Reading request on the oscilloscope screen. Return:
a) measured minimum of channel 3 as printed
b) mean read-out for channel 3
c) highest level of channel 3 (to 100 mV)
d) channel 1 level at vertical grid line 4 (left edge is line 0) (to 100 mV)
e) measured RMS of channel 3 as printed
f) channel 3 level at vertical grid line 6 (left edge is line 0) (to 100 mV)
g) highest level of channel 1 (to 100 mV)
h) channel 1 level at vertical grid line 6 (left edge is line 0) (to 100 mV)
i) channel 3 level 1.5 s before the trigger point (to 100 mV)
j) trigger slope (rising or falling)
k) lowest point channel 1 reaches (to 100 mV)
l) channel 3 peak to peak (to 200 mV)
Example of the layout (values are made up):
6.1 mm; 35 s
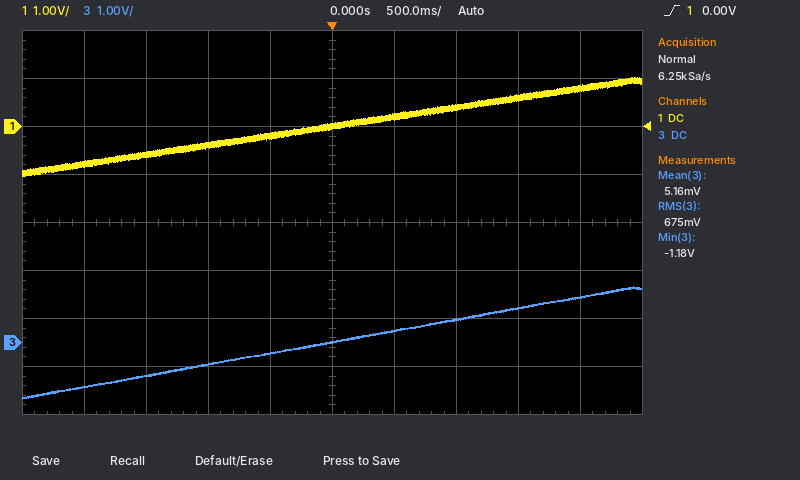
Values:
-1.18 V; 5.16 mV; 1.2 V; -200 mV; 675 mV; 200 mV; 1.0 V; 200 mV; -700 mV; rising; -1.0 V; 2.4 V
